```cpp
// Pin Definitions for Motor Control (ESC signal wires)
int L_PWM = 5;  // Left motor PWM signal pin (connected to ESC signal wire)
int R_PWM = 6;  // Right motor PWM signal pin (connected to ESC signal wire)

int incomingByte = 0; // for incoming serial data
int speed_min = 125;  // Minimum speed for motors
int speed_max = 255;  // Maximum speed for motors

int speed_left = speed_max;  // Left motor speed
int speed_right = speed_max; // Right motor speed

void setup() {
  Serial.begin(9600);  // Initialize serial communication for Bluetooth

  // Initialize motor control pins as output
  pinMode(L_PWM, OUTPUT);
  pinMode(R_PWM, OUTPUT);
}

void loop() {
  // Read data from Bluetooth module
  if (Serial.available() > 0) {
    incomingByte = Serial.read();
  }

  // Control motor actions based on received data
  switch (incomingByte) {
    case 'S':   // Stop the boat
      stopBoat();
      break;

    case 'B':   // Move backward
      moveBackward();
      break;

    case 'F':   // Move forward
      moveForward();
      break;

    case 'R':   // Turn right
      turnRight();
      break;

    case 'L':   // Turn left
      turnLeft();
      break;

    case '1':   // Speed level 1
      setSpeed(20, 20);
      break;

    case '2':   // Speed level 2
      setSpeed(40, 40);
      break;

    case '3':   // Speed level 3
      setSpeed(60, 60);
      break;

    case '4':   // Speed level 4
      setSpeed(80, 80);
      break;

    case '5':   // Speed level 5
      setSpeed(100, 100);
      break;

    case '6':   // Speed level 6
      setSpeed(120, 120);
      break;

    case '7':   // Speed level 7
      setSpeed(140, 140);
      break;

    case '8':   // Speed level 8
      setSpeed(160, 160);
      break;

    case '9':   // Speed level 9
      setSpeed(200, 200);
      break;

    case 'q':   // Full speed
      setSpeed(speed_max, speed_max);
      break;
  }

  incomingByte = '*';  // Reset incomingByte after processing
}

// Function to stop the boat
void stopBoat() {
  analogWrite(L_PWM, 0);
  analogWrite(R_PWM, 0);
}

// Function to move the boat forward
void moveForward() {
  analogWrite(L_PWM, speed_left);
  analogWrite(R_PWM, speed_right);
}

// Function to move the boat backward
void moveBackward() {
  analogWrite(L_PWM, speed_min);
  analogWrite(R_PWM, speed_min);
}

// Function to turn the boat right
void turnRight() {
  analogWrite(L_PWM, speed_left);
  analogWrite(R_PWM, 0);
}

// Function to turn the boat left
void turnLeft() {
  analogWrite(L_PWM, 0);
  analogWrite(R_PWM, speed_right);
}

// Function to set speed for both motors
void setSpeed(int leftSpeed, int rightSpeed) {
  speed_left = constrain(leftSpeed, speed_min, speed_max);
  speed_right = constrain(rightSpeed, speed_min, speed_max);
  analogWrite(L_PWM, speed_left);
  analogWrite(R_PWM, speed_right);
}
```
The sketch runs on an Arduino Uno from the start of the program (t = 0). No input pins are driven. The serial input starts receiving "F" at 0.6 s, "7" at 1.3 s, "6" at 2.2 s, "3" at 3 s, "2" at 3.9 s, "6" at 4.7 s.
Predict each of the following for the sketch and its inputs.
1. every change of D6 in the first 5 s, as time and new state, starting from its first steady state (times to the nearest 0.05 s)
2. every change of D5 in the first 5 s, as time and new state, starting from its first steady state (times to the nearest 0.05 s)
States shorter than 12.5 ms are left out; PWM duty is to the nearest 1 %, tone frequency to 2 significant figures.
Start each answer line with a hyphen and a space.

- 0 s low; 0.6 s high; 1.3 s PWM 55 %; 2.2 s PWM 49 %
- 0 s low; 0.6 s high; 1.3 s PWM 55 %; 2.2 s PWM 49 %
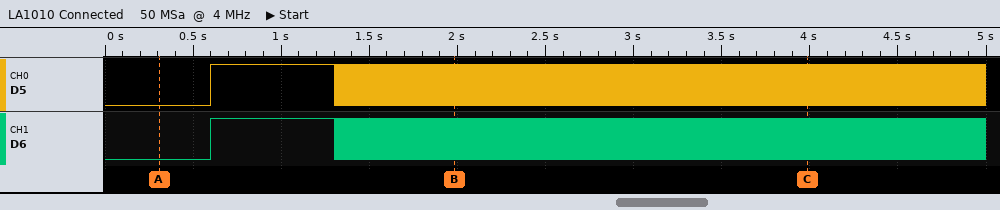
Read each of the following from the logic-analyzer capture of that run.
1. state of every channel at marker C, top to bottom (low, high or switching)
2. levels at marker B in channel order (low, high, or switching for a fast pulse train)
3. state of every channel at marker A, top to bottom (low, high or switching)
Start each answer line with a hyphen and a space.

- D5 switching, D6 switching
- D5 switching, D6 switching
- D5 low, D6 low
